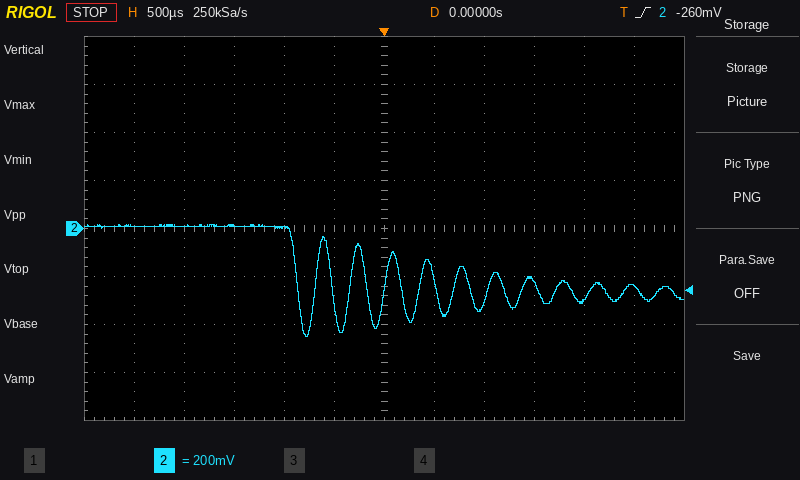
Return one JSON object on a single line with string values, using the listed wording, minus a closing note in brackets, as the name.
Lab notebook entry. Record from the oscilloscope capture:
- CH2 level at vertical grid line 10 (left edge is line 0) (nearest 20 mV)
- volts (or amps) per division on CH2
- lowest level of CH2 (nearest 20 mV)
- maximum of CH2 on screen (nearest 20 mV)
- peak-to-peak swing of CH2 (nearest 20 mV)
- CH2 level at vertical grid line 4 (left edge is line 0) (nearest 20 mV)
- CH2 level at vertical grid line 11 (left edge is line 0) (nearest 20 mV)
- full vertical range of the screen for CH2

{"CH2 level at vertical grid line 10 (left edge is line 0)": "-300 mV", "volts (or amps) per division on CH2": "200 mV", "lowest level of CH2": "-440 mV", "maximum of CH2 on screen": "20 mV", "peak-to-peak swing of CH2": "460 mV", "CH2 level at vertical grid line 4 (left edge is line 0)": "0 mV", "CH2 level at vertical grid line 11 (left edge is line 0)": "-240 mV", "full vertical range of the screen for CH2": "1.6 V"}
